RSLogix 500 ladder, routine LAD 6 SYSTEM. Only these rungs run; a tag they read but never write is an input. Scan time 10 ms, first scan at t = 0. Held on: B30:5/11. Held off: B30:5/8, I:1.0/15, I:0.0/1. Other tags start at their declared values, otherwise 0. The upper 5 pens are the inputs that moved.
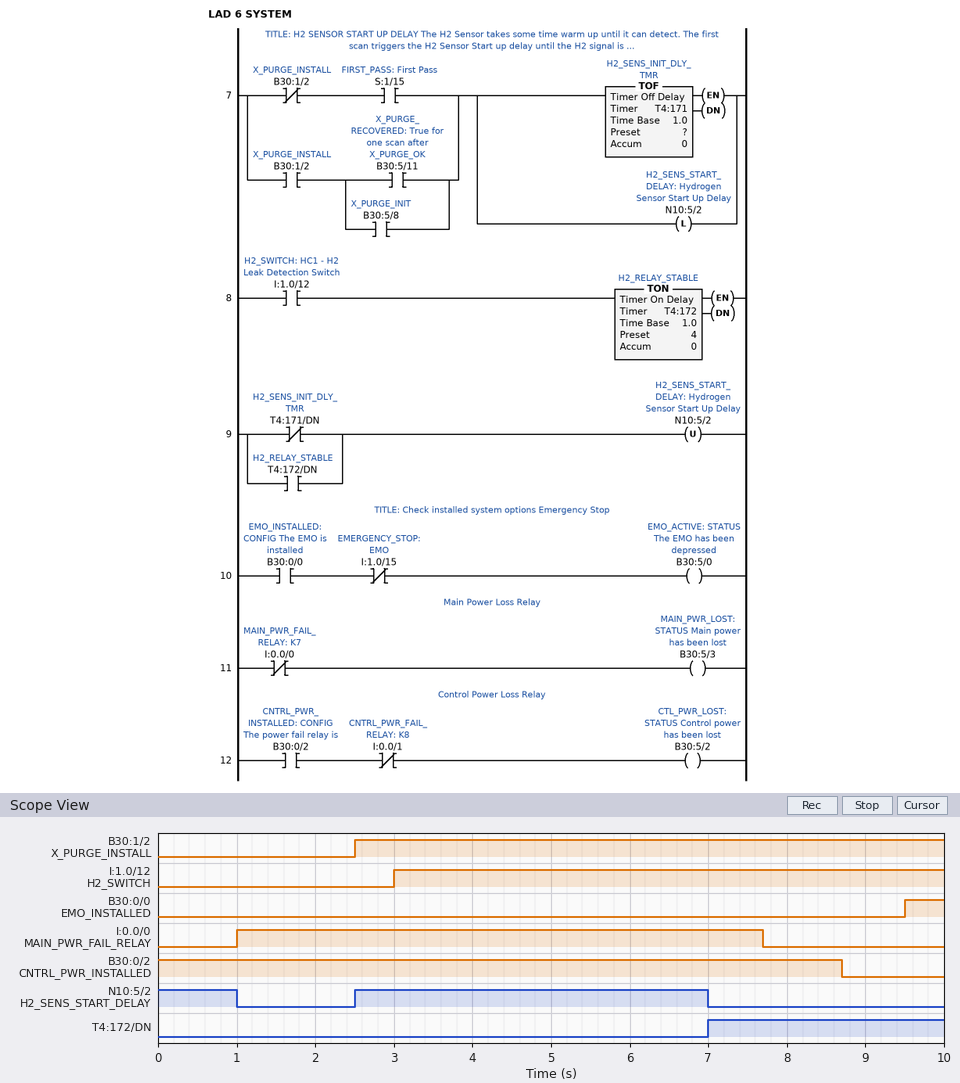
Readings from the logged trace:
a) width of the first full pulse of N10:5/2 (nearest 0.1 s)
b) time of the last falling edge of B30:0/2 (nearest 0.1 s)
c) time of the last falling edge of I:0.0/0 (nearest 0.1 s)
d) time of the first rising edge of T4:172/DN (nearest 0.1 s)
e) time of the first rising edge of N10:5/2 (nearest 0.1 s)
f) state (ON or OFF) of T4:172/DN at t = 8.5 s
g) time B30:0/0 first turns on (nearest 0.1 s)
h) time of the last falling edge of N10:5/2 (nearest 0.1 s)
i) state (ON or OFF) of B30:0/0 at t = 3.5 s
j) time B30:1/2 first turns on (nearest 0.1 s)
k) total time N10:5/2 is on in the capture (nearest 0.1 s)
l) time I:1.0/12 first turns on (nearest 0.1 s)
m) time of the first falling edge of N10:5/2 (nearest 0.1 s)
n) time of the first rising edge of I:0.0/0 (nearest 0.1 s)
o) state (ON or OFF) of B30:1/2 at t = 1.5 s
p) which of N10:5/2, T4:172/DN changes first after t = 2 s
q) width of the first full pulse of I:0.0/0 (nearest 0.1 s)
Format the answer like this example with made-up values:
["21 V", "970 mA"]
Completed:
["4.5 s", "8.7 s", "7.7 s", "7.0 s", "2.5 s", "ON", "9.5 s", "7.0 s", "OFF", "2.5 s", "5.5 s", "3.0 s", "1.0 s", "1.0 s", "OFF", "N10:5/2", "6.7 s"]
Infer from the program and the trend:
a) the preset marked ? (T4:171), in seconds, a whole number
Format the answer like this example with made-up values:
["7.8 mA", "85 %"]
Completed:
["1 s"]
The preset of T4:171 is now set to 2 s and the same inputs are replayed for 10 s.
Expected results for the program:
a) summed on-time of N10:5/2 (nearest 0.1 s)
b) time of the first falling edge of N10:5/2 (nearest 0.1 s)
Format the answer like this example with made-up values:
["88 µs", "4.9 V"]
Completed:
["6.5 s", "2.0 s"]
